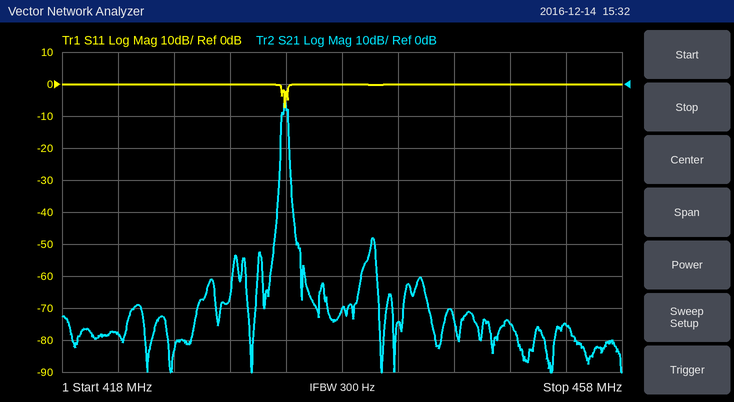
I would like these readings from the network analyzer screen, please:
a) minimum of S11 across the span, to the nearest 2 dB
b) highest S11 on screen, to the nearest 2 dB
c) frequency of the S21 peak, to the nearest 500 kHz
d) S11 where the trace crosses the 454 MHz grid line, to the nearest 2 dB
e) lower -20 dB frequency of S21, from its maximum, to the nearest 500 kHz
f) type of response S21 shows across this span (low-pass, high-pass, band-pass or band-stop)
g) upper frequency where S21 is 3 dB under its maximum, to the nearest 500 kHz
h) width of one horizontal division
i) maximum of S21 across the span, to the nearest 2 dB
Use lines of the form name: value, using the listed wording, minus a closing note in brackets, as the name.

minimum of S11 across the span, to the nearest 2 dB: -8 dB
highest S11 on screen, to the nearest 2 dB: 0 dB
frequency of the S21 peak, to the nearest 500 kHz: 434.0 MHz
S11 where the trace crosses the 454 MHz grid line, to the nearest 2 dB: 0 dB
lower -20 dB frequency of S21, from its maximum, to the nearest 500 kHz: 433.5 MHz
type of response S21 shows across this span: band-pass
upper frequency where S21 is 3 dB under its maximum, to the nearest 500 kHz: 434.0 MHz
width of one horizontal division: 4 MHz
maximum of S21 across the span, to the nearest 2 dB: -6 dB
